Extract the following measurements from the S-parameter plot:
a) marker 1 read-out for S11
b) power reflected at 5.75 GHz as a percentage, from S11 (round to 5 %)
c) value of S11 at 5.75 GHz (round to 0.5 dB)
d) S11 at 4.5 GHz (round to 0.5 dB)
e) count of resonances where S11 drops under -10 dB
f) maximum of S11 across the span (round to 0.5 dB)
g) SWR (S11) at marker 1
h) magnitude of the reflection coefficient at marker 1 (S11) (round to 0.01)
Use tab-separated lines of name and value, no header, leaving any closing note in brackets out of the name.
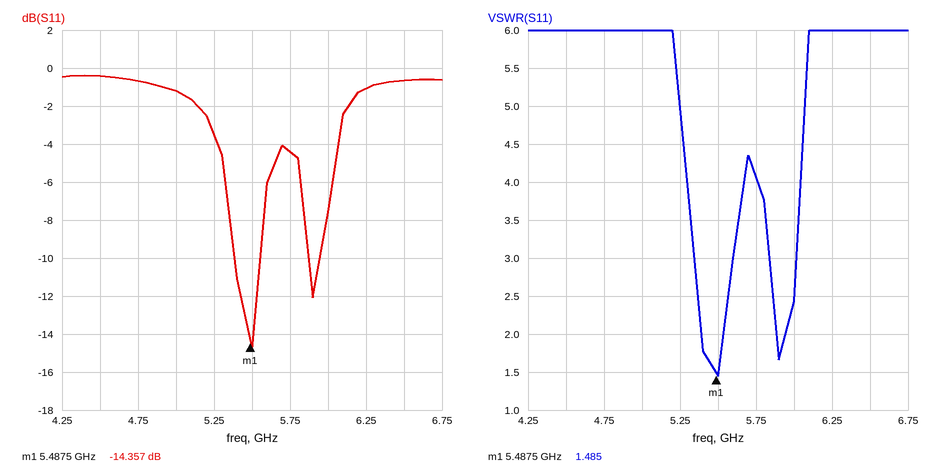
marker 1 read-out for S11	-14.357 dB
power reflected at 5.75 GHz as a percentage, from S11	35 %
value of S11 at 5.75 GHz	-4.5 dB
S11 at 4.5 GHz	-0.5 dB
count of resonances where S11 drops under -10 dB	2
maximum of S11 across the span	-0.5 dB
SWR (S11) at marker 1	1.485
magnitude of the reflection coefficient at marker 1 (S11)	0.19
